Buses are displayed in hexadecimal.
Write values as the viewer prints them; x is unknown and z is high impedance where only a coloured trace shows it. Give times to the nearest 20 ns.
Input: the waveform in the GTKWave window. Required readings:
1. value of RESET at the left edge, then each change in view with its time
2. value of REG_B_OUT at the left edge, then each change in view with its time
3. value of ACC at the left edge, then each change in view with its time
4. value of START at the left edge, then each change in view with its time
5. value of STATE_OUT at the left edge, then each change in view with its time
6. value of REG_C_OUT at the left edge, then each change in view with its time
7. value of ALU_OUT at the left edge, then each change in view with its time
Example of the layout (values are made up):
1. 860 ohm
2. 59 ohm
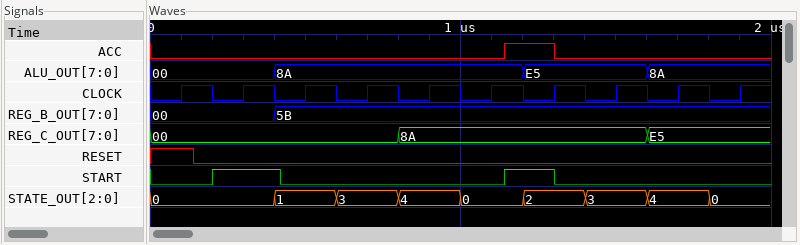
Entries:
1. 1, 0 at 140 ns
2. 00, 5B at 400 ns
3. 0, 1 at 1140 ns, 0 at 1300 ns
4. 0, 1 at 200 ns, 0 at 420 ns, 1 at 1140 ns, 0 at 1300 ns
5. 0, 1 at 400 ns, 3 at 600 ns, 4 at 800 ns, 0 at 1000 ns, 2 at 1200 ns, 3 at 1400 ns, 4 at 1600 ns, 0 at 1800 ns
6. 00, 8A at 800 ns, E5 at 1600 ns
7. 00, 8A at 400 ns, E5 at 1200 ns, 8A at 1600 ns
